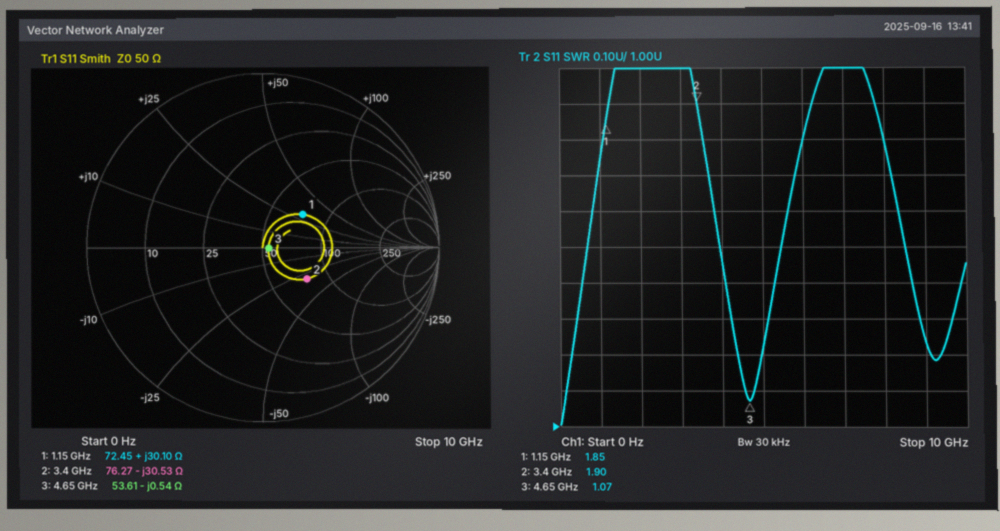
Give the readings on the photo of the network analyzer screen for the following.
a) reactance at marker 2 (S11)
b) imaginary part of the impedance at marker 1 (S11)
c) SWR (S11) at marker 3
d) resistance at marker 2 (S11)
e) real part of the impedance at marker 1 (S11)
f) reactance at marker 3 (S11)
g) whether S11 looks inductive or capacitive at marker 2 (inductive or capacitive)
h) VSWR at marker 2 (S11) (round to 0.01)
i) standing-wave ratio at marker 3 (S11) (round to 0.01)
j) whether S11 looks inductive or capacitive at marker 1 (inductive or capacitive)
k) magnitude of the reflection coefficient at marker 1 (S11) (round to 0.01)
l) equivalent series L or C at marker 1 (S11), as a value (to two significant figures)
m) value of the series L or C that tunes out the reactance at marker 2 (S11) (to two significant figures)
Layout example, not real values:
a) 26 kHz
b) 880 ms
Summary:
a) -30.53 Ω
b) +30.10 Ω
c) 1.07
d) 76.27 Ω
e) 72.45 Ω
f) -0.54 Ω
g) capacitive
h) 1.90
i) 1.07
j) inductive
k) 0.30
l) 4.2 nH
m) 1.4 nH
